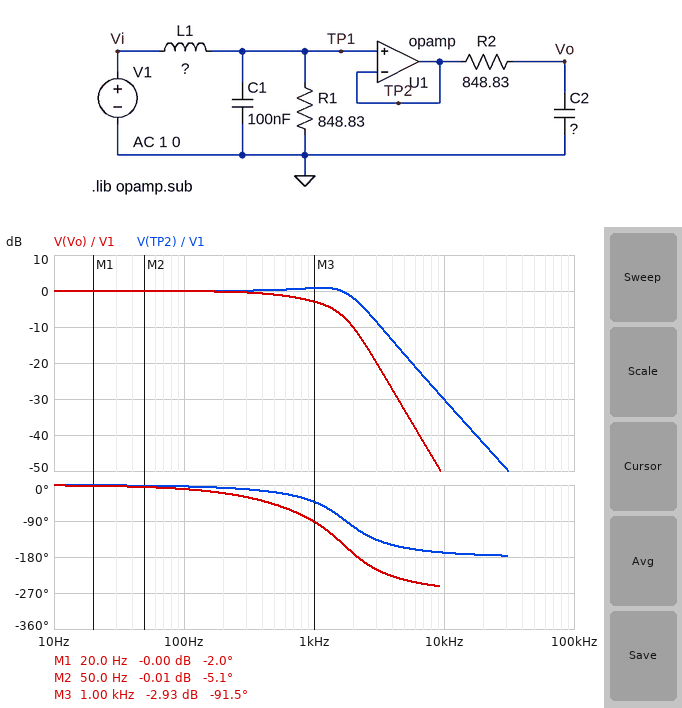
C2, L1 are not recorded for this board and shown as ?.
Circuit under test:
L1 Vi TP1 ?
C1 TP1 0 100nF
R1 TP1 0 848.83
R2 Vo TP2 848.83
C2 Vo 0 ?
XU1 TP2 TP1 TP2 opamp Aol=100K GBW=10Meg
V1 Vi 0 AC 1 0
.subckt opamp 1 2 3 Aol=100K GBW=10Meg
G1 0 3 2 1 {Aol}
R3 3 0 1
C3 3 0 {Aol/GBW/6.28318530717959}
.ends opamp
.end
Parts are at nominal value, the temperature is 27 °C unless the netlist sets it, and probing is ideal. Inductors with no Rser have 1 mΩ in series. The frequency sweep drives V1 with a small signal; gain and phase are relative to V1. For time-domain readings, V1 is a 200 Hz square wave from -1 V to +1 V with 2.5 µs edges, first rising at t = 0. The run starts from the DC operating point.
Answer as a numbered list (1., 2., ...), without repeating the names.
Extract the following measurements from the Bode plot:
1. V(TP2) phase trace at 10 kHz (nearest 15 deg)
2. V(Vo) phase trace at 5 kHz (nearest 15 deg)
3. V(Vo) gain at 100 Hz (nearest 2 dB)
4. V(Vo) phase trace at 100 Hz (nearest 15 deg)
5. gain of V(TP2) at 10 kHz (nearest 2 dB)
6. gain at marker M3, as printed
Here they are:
1. -165 deg
2. -240 deg
3. 0 dB
4. -15 deg
5. -30 dB
6. -2.93 dB
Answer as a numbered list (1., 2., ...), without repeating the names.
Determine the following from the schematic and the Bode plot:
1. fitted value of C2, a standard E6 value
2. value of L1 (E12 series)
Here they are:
1. 220 nF
2. 82 mH
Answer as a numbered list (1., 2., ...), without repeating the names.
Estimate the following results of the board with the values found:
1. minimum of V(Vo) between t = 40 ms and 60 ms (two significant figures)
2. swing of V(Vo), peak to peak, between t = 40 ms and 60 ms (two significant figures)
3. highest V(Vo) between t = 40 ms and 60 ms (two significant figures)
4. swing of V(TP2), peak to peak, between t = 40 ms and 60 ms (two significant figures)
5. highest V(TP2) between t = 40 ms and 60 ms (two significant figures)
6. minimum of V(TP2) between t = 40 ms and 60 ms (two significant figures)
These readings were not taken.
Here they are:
1. -1.0 V
2. 2.0 V
3. 1.0 V
4. 2.6 V
5. 1.3 V
6. -1.3 V
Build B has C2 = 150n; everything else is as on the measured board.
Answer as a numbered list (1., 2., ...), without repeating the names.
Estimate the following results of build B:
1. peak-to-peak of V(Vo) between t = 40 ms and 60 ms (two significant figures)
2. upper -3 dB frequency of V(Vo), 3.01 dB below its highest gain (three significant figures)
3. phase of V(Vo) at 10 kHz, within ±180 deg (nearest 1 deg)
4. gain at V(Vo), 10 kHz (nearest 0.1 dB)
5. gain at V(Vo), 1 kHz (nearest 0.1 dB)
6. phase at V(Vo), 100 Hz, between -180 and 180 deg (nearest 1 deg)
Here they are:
1. 2.1 V
2. 1.43 kHz
3. 108 deg
4. -48.2 dB
5. -1.3 dB
6. -8 deg
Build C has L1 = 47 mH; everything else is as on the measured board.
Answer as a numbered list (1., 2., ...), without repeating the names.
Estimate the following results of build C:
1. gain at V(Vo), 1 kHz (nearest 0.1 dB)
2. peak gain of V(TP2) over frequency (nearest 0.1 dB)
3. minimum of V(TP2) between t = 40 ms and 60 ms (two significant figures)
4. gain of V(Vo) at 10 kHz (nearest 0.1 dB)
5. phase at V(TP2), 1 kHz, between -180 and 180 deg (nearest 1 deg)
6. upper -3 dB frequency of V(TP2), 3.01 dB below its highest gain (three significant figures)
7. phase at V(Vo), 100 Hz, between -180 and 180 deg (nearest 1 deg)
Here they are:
1. -2.7 dB
2. 2.6 dB
3. -1.5 V
4. -46.5 dB
5. -23 deg
6. 2.76 kHz
7. -9 deg
